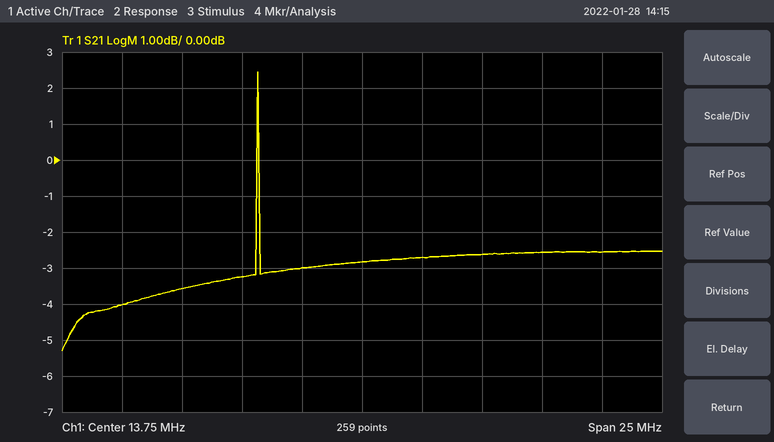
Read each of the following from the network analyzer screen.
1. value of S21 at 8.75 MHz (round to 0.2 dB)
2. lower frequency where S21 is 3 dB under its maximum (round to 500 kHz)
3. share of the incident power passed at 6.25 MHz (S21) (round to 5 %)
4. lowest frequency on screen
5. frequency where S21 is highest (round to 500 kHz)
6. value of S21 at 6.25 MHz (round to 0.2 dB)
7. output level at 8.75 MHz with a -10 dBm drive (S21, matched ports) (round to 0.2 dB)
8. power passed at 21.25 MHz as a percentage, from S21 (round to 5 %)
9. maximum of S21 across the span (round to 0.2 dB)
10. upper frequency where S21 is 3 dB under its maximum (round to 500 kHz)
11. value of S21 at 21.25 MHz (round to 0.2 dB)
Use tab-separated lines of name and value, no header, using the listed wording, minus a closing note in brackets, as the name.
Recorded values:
value of S21 at 8.75 MHz	-3.2 dB
lower frequency where S21 is 3 dB under its maximum	9.5 MHz
share of the incident power passed at 6.25 MHz (S21)	45 %
lowest frequency on screen	1.25 MHz
frequency where S21 is highest	9.5 MHz
value of S21 at 6.25 MHz	-3.6 dB
output level at 8.75 MHz with a -10 dBm drive (S21, matched ports)	-13.2 dBm
power passed at 21.25 MHz as a percentage, from S21	55 %
maximum of S21 across the span	2.4 dB
upper frequency where S21 is 3 dB under its maximum	9.5 MHz
value of S21 at 21.25 MHz	-2.6 dB
